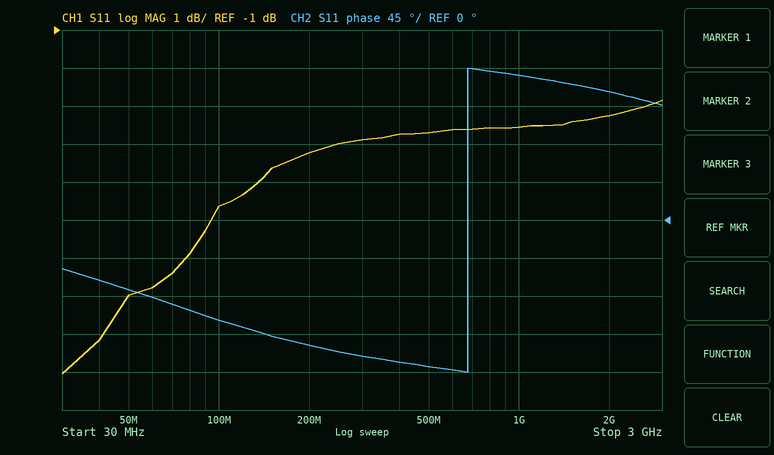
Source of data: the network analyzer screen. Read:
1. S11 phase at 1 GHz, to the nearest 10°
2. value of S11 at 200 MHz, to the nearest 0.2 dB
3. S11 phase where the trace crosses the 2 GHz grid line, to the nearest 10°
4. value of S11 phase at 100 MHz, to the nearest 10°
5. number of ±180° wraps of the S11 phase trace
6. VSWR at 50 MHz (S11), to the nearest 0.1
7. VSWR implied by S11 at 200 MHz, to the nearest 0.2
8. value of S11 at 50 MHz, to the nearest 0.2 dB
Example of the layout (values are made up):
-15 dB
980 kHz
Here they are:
170°
-4.2 dB
150°
-120°
1
2.3
4.2
-8.0 dB
